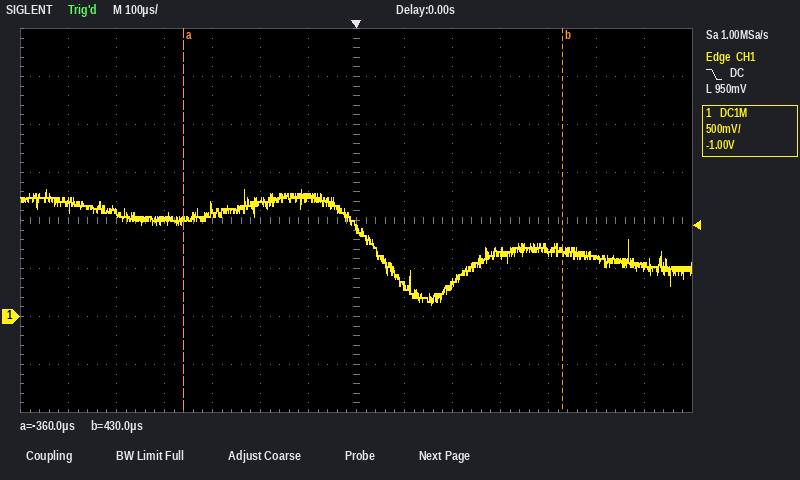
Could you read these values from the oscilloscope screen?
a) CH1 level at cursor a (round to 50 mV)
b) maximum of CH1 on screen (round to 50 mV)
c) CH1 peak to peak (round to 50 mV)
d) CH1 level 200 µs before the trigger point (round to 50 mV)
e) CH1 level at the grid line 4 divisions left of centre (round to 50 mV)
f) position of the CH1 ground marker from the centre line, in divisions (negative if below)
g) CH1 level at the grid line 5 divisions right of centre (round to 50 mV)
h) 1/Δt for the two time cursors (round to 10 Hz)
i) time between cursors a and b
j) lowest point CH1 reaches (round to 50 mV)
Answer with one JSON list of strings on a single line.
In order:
["1.00 V", "1.30 V", "1.20 V", "1.20 V", "1.00 V", "-2.0 div", "600 mV", "1.27 kHz", "790 µs", "100 mV"]
